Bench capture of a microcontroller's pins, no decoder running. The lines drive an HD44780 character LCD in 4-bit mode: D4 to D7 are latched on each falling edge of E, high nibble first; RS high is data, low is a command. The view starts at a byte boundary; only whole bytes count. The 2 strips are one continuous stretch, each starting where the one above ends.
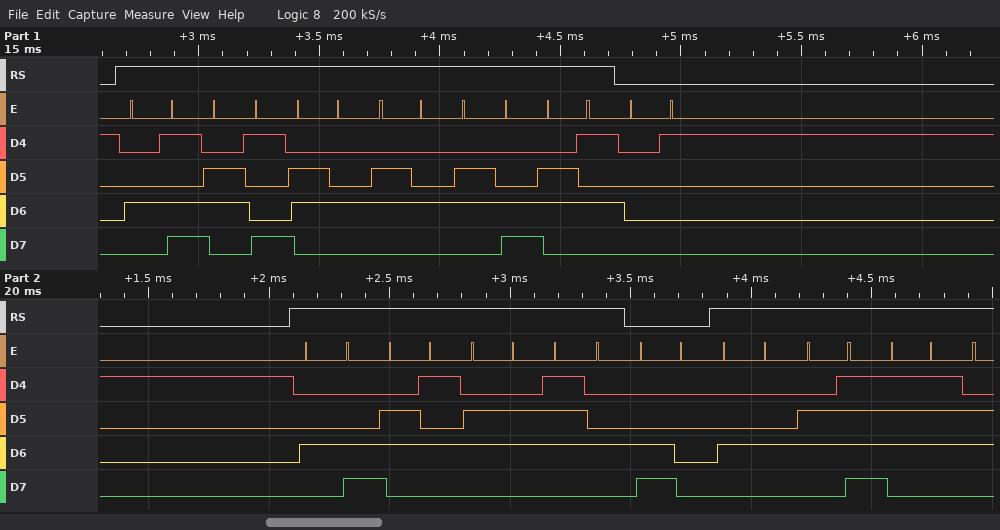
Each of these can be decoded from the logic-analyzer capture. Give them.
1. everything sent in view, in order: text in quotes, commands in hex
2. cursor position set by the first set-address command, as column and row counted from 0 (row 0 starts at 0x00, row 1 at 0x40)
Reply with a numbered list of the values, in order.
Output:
1. "Middle" 0x01 "Left" 0xC0 "Dow"
2. column 0, row 1
